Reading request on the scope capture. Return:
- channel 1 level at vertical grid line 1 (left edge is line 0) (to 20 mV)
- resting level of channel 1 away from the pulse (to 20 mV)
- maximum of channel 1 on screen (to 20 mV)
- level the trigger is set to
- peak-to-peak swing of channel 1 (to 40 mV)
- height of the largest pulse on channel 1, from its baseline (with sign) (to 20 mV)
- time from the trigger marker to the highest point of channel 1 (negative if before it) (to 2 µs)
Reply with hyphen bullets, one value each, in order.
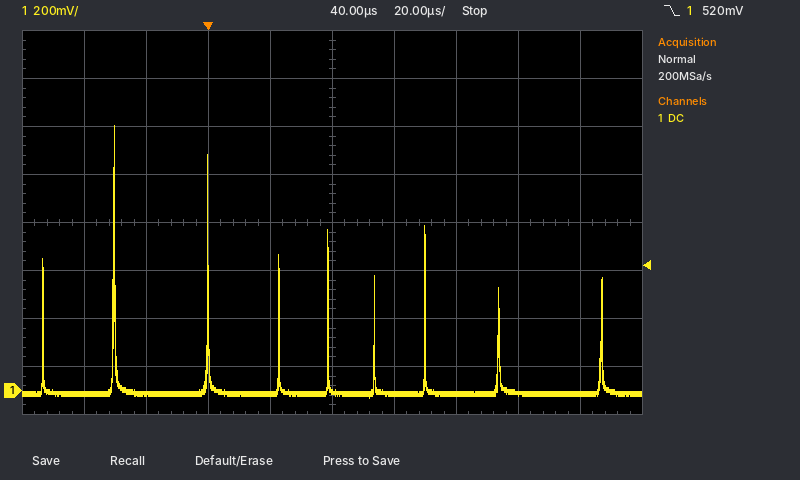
- -20 mV
- -20 mV
- 1.10 V
- 520 mV
- 1.12 V
- +1.12 V
- -30 µs
